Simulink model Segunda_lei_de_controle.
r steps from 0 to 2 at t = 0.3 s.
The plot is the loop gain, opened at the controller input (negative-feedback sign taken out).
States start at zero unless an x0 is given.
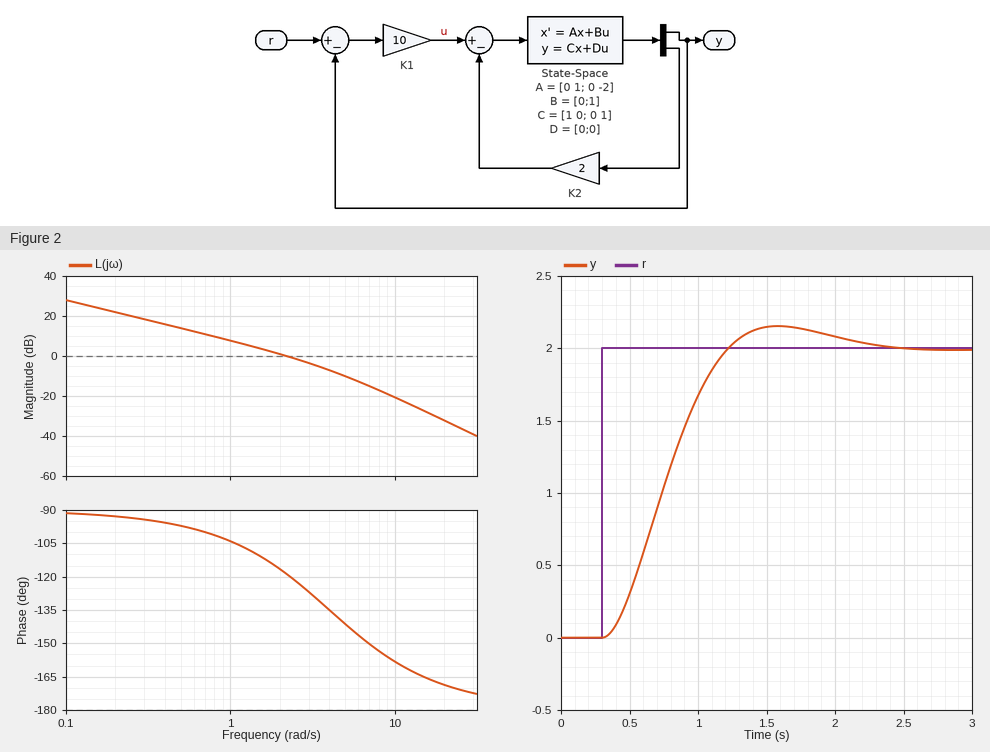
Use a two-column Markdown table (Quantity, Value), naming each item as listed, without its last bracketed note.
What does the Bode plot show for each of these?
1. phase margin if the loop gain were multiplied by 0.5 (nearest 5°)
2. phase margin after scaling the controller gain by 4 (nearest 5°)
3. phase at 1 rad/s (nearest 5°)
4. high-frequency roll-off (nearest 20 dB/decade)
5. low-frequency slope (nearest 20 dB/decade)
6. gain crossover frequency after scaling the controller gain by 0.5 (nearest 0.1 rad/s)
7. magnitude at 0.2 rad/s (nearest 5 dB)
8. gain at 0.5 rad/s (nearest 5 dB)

| Quantity | Value |
|---|---|
| phase margin if the loop gain were multiplied by 0.5 | 75° |
| phase margin after scaling the controller gain by 4 | 35° |
| phase at 1 rad/s | -105° |
| high-frequency roll-off | -40 dB/decade |
| low-frequency slope | -20 dB/decade |
| gain crossover frequency after scaling the controller gain by 0.5 | 1.2 rad/s |
| magnitude at 0.2 rad/s | 20 dB |
| gain at 0.5 rad/s | 15 dB |
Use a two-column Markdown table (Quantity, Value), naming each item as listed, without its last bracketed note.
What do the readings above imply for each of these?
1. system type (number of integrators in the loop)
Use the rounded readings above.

| Quantity | Value |
|---|---|
| system type | 1 |
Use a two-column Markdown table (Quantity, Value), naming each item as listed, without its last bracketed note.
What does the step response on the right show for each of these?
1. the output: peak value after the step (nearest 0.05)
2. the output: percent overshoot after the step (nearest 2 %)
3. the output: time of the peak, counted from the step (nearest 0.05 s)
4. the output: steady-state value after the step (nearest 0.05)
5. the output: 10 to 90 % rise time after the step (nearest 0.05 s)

| Quantity | Value |
|---|---|
| the output: peak value after the step | 2.15 |
| the output: percent overshoot after the step | 8 % |
| the output: time of the peak, counted from the step | 1.30 s |
| the output: steady-state value after the step | 2.00 |
| the output: 10 to 90 % rise time after the step | 0.60 s |
